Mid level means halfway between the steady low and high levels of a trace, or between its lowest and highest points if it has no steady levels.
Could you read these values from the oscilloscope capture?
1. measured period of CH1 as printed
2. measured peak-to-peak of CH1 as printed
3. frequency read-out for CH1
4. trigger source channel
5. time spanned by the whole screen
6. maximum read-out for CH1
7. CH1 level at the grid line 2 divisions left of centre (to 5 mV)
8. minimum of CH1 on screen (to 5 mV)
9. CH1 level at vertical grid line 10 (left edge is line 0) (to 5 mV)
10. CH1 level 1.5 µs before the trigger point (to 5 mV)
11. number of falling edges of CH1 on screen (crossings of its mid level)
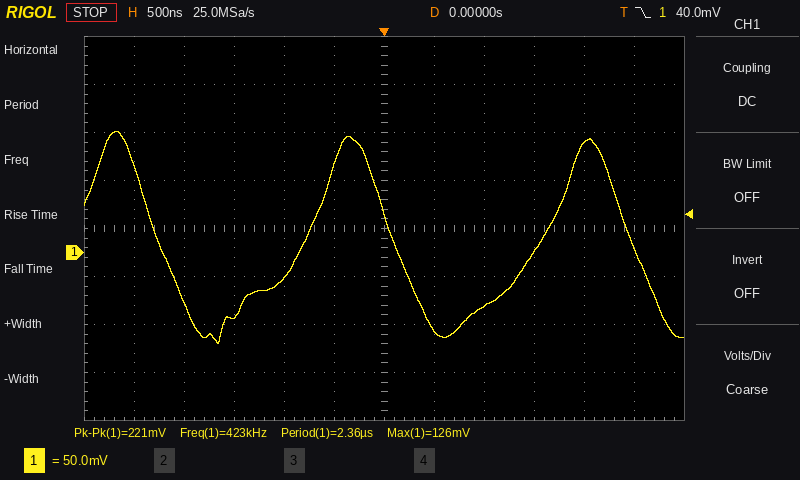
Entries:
2.36 µs
221 mV
423 kHz
CH1
6 µs
126 mV
-25 mV
-95 mV
115 mV
-65 mV
3
